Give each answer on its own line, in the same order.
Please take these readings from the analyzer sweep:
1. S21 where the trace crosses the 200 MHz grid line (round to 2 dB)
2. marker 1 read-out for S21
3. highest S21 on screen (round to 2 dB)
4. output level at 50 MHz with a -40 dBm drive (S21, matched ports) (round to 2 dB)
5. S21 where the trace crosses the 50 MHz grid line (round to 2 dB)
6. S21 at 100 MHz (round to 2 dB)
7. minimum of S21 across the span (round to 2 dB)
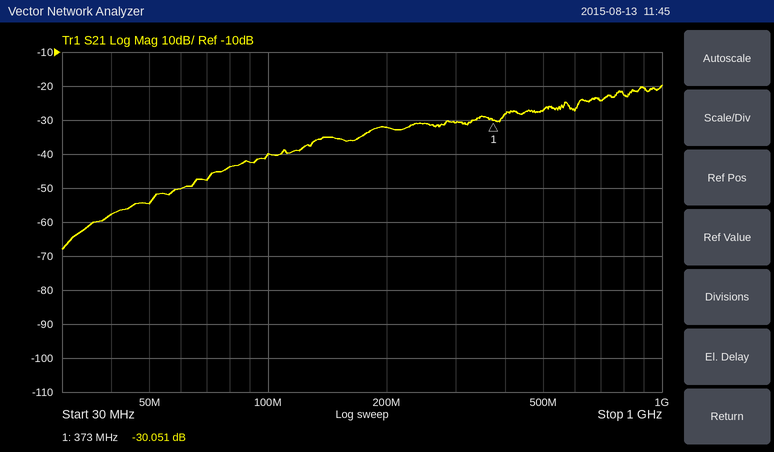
-32 dB
-30.051 dB
-20 dB
-94 dBm
-54 dB
-40 dB
-68 dB
